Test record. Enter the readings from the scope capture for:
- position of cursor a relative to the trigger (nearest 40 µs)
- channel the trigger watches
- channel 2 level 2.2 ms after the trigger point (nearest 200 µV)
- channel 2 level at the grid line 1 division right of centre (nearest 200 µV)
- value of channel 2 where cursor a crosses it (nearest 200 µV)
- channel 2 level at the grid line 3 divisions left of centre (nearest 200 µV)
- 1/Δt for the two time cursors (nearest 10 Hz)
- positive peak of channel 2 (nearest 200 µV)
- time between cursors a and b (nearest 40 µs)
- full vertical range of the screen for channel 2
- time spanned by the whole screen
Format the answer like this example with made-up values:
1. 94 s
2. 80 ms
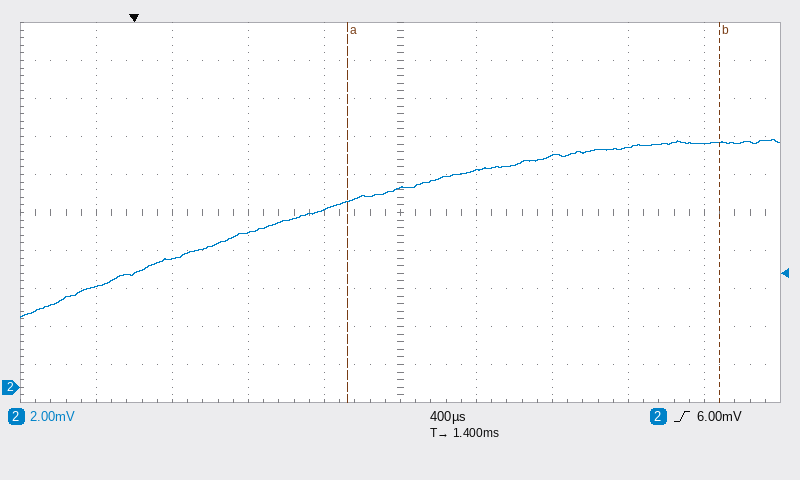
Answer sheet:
1. +1.12 ms
2. channel 2
3. 12.2 mV
4. 11.4 mV
5. 9.8 mV
6. 6.8 mV
7. 510 Hz
8. 13.0 mV
9. 1.96 ms
10. 20 mV
11. 4 ms
